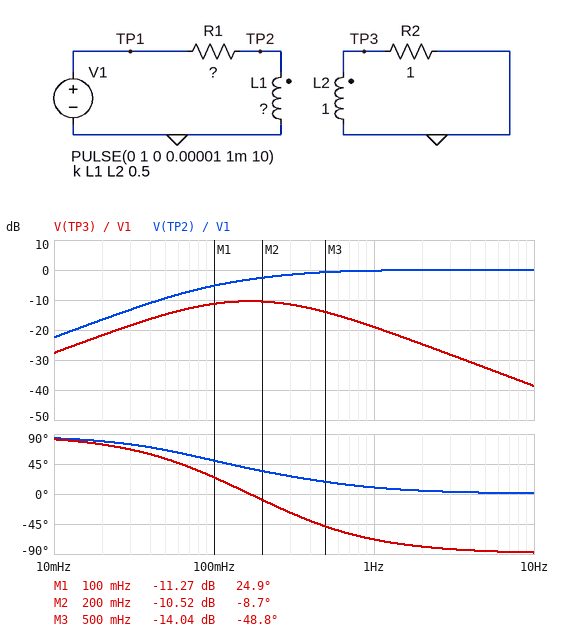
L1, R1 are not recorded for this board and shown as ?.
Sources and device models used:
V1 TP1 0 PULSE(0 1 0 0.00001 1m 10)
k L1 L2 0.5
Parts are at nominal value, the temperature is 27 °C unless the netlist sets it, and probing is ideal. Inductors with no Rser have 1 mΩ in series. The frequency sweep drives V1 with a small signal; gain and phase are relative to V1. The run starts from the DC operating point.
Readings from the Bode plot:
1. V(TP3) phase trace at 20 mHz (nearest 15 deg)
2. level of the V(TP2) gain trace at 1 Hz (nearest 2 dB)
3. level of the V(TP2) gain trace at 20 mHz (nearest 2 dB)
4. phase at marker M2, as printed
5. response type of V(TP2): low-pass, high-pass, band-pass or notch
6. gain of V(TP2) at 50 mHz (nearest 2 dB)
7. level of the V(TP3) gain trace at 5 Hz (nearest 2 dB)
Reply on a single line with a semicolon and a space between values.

75 deg; 0 dB; -16 dB; -8.7 deg; high-pass; -10 dB; -32 dB
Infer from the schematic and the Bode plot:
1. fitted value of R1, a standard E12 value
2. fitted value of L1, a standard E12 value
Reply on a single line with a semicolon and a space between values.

0.68 Ω; 820 mH
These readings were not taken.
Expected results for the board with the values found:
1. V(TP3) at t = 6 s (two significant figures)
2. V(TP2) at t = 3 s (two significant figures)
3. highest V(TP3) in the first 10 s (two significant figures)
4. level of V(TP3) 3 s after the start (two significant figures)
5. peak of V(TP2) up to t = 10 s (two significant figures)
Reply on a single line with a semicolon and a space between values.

16 mV; 100 mV; 230 mV; 95 mV; 1.0 V
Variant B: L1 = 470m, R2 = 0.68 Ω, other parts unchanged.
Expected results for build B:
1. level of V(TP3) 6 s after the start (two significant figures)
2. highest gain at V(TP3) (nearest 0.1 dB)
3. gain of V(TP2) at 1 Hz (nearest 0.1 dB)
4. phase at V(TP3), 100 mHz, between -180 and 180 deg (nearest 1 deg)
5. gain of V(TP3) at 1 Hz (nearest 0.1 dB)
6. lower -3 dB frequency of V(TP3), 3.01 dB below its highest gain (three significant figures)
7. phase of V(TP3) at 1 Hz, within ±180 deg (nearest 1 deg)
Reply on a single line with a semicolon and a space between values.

12 mV; -12.7 dB; -0.5 dB; 27 deg; -20.1 dB; 64.5 mHz; -65 deg
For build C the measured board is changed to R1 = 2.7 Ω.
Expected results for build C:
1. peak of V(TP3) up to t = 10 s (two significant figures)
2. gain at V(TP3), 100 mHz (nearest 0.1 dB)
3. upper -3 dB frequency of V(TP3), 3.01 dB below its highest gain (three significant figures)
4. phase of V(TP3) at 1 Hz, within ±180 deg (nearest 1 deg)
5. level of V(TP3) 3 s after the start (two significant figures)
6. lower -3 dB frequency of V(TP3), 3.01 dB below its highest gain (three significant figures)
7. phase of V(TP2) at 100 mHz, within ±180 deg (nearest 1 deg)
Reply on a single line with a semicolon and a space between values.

100 mV; -21.3 dB; 1.02 Hz; -44 deg; 12 mV; 109 mHz; 73 deg
